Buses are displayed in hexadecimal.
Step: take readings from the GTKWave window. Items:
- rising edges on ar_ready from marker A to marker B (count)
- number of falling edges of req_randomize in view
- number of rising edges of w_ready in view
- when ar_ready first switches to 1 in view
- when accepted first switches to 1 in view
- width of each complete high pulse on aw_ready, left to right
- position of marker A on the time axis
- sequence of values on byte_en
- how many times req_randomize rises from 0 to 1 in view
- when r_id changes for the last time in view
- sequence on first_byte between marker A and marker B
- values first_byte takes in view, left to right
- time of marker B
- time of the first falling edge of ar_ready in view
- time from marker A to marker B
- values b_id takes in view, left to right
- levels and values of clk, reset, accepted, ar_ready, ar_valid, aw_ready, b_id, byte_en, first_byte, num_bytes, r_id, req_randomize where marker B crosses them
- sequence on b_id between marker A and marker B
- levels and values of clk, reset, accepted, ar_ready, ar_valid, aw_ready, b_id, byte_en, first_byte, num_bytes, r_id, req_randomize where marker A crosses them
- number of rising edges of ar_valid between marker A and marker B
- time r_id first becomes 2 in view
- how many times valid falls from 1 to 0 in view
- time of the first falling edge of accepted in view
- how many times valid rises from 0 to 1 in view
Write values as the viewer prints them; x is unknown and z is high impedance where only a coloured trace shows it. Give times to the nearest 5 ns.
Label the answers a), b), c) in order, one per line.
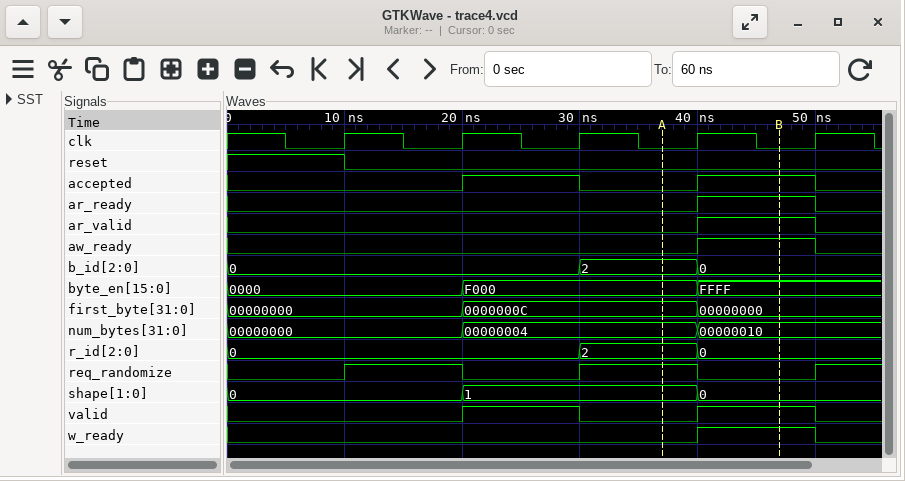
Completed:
a) 1
b) 2
c) 1
d) 40 ns
e) 20 ns
f) 10 ns
g) 35 ns
h) 0000, F000, FFFF
i) 3
j) 40 ns
k) 0000000C, 00000000
l) 00000000, 0000000C, 00000000
m) 45 ns
n) 50 ns
o) 10 ns
p) 0, 2, 0
q) clk=0, reset=0, accepted=1, ar_ready=1, ar_valid=1, aw_ready=1, b_id=0, byte_en=FFFF, first_byte=00000000, num_bytes=00000010, r_id=0, req_randomize=0
r) 2, 0
s) clk=0, reset=0, accepted=0, ar_ready=0, ar_valid=0, aw_ready=0, b_id=2, byte_en=F000, first_byte=0000000C, num_bytes=00000004, r_id=2, req_randomize=1
t) 1
u) 30 ns
v) 2
w) 30 ns
x) 2
